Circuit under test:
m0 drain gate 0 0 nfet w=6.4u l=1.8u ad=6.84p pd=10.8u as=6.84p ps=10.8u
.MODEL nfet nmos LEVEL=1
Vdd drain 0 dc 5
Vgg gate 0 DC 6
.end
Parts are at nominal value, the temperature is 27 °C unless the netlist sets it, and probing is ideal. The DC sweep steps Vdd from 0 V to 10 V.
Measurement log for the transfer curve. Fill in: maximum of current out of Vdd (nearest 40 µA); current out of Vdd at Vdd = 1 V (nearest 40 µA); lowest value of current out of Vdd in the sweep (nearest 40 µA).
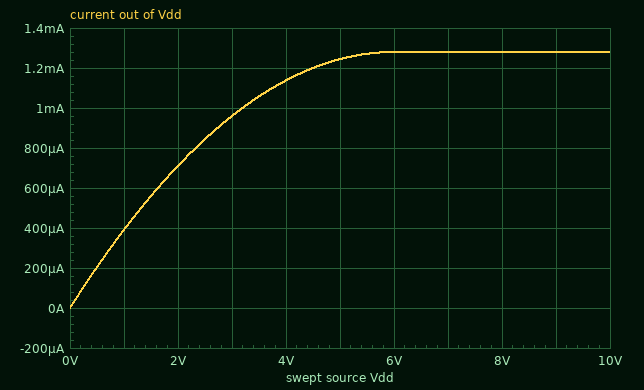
1.28 mA
400 µA
0 A
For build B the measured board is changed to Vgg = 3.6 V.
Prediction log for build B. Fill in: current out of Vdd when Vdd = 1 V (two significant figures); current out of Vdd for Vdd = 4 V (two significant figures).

220 µA
460 µA
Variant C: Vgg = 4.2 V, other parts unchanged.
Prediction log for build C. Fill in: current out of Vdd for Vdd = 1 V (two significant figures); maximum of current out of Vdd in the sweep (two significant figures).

260 µA
630 µA
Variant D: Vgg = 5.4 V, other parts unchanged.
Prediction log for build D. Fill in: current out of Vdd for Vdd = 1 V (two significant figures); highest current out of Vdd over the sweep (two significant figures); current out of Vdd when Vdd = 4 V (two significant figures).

350 µA
1.0 mA
970 µA
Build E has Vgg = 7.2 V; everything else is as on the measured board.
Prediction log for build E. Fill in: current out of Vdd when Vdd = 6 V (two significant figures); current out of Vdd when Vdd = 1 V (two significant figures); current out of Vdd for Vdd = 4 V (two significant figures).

1.8 mA
480 µA
1.5 mA
